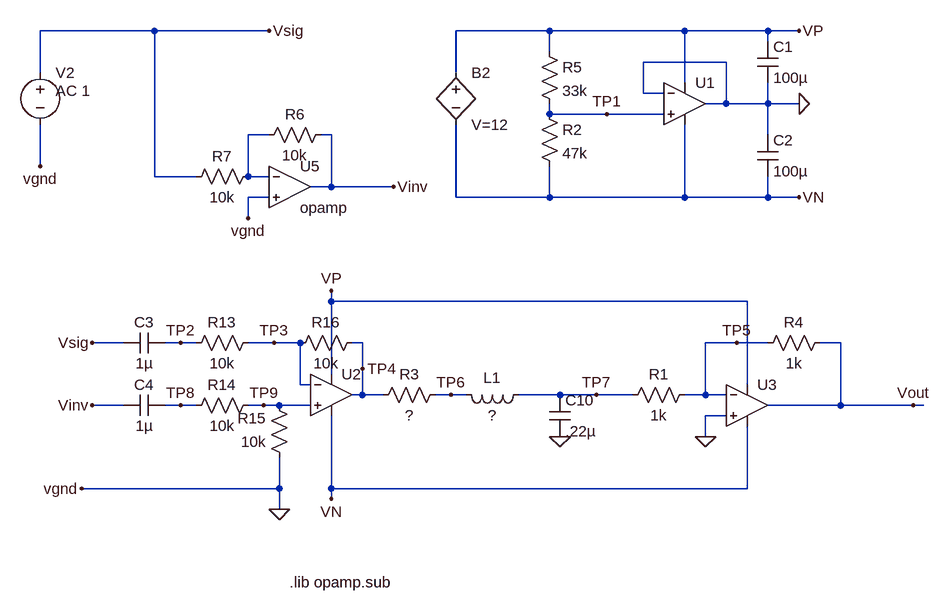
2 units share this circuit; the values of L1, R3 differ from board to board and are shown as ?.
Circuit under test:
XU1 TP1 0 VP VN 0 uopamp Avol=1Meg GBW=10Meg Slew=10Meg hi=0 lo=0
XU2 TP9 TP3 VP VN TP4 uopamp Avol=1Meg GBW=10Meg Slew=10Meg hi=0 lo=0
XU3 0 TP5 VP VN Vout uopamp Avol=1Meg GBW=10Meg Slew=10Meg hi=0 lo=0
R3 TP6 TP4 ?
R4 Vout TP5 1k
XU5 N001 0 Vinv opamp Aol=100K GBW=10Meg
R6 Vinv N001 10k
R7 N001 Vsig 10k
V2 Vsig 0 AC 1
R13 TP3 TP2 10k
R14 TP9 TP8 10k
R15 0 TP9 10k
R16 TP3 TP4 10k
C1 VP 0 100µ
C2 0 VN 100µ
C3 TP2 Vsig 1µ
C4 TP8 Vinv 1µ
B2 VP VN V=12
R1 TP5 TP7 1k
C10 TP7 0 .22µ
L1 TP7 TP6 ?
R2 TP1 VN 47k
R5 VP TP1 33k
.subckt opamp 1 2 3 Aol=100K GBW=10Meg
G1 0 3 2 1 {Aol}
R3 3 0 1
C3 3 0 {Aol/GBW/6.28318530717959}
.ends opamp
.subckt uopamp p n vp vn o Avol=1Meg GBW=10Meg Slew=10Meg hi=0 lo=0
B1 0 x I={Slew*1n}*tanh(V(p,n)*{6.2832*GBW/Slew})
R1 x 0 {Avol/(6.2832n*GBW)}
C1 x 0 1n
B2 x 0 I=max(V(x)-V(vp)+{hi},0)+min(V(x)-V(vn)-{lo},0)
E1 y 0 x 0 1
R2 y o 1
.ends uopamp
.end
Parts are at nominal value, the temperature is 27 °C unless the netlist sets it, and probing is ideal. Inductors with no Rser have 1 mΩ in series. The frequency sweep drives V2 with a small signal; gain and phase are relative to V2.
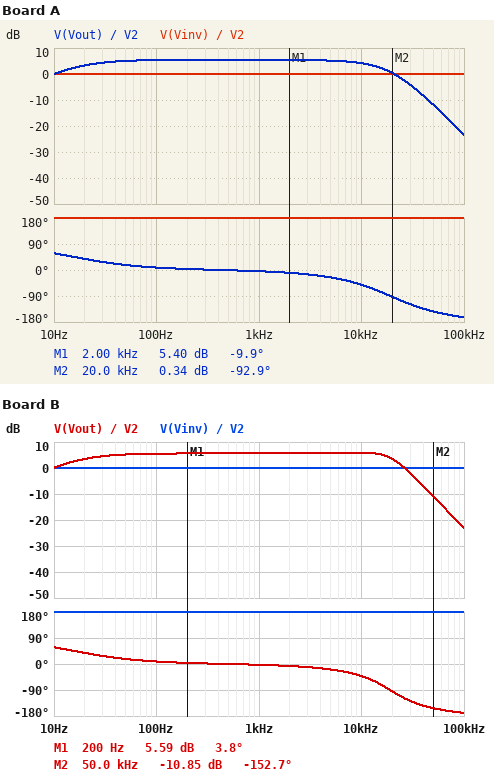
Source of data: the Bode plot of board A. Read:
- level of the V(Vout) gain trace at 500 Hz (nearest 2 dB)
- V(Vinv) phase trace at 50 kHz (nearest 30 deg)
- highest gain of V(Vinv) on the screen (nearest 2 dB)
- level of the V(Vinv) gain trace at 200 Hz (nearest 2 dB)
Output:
6 dB
180 deg
0 dB
0 dB
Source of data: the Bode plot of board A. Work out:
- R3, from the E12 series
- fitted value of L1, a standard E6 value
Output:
68 Ω
330 µH
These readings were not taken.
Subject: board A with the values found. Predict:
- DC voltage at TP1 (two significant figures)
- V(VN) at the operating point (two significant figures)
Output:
3.5 V
-3.5 V
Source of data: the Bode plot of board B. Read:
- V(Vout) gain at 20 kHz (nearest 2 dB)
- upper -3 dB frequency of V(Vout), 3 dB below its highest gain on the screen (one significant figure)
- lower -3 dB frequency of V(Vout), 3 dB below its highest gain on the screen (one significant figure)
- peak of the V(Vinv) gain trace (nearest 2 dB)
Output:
4 dB
20 kHz
20 Hz
0 dB
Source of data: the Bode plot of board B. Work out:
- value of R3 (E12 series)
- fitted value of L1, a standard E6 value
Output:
47 Ω
330 µH
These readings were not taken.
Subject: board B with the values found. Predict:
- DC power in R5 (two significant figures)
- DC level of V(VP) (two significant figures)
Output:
740 µW
8.5 V
